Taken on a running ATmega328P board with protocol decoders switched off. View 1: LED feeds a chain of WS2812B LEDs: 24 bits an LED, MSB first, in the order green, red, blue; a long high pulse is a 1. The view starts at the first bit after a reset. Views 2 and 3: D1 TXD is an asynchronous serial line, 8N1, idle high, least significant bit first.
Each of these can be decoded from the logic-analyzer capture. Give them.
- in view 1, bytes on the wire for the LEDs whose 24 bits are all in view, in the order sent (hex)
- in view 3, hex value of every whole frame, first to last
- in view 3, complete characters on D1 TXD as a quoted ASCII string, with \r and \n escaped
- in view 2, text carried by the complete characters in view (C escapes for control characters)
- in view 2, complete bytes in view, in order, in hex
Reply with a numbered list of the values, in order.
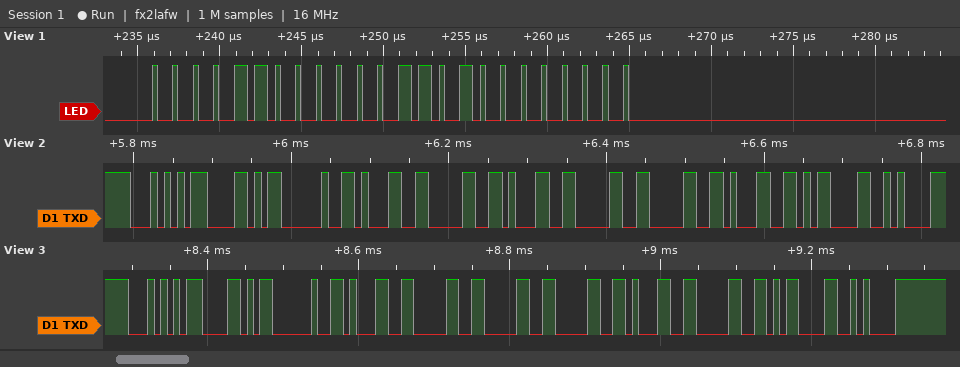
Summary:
1. 0C 0D 00
2. 54 58 20 31 30 30 30 31 30 0D 0A
3. "TX 100010\r\n"
4. "TX 101001\r\n"
5. 54 58 20 31 30 31 30 30 31 0D 0A
